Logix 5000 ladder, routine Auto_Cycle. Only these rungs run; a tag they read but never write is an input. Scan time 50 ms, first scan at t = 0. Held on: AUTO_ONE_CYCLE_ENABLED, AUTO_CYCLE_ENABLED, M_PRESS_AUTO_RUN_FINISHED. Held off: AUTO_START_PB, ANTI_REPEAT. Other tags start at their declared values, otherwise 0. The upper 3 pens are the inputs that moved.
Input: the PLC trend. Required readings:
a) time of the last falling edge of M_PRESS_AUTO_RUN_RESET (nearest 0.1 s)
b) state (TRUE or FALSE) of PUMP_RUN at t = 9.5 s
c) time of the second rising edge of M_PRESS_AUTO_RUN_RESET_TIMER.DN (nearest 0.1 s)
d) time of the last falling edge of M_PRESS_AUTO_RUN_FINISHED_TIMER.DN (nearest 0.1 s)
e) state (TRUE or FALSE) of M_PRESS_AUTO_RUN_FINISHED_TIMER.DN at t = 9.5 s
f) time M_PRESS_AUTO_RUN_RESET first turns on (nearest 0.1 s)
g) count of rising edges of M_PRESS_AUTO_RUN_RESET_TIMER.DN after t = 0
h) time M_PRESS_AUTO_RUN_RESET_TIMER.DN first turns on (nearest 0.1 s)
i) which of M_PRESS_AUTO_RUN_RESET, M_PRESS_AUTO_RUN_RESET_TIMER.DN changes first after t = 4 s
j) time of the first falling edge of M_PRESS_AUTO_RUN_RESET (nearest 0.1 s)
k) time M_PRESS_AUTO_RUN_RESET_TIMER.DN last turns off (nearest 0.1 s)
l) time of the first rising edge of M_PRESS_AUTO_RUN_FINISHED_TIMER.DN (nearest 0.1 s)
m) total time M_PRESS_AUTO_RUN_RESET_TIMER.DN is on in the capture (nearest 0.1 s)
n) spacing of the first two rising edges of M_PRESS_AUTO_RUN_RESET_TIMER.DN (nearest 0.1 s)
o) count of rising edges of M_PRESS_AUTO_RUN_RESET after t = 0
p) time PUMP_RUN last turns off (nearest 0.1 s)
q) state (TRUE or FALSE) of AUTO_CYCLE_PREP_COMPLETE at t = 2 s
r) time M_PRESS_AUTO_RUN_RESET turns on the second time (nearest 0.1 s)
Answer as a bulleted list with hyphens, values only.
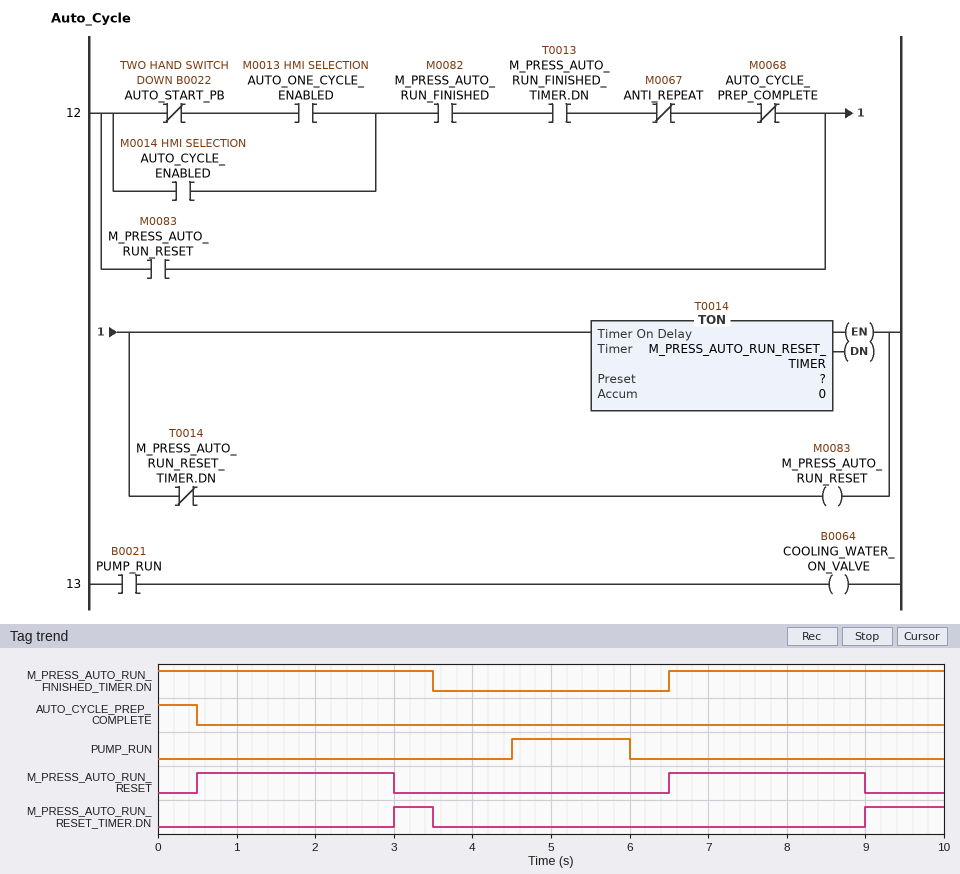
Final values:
- 9.0 s
- FALSE
- 9.0 s
- 3.5 s
- TRUE
- 0.5 s
- 2
- 3.0 s
- M_PRESS_AUTO_RUN_RESET
- 3.0 s
- 3.5 s
- 6.5 s
- 1.5 s
- 6.0 s
- 2
- 6.0 s
- FALSE
- 6.5 s
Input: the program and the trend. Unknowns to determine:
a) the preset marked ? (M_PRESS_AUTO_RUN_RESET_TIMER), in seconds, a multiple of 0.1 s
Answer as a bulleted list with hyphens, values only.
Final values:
- 2.5 s
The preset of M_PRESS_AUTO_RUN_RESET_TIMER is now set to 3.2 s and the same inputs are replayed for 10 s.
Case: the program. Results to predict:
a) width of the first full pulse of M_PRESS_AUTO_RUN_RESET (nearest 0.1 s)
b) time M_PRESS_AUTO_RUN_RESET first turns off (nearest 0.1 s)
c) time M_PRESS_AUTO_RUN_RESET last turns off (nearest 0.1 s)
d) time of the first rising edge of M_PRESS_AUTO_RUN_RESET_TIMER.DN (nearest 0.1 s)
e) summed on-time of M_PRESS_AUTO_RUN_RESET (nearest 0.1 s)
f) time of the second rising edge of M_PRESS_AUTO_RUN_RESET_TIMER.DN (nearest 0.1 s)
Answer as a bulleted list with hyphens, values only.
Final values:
- 3.2 s
- 3.7 s
- 9.7 s
- 3.7 s
- 6.4 s
- 9.7 s
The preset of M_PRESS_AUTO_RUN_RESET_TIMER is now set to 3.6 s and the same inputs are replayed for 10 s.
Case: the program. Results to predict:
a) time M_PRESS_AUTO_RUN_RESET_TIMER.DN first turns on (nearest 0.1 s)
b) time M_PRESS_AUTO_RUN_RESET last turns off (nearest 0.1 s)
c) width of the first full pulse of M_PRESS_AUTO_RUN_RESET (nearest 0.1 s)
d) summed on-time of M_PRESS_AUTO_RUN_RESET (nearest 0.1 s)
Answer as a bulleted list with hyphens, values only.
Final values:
- 4.1 s
- 4.1 s
- 3.6 s
- 7.1 s
